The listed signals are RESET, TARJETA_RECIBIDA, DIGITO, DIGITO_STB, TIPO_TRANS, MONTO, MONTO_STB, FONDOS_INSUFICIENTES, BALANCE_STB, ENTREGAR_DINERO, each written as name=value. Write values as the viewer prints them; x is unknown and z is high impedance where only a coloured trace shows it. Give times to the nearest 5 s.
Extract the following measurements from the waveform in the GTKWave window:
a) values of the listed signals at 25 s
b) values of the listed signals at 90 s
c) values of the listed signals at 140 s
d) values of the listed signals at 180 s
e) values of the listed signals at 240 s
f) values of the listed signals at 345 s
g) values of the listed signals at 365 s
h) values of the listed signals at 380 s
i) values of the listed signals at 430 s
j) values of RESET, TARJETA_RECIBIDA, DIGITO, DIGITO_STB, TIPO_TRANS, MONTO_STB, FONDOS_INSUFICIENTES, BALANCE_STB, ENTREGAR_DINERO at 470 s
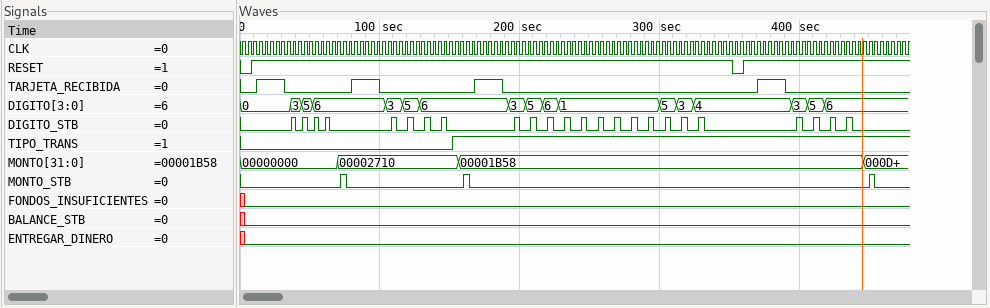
RESET=1, TARJETA_RECIBIDA=1, DIGITO=0, DIGITO_STB=0, TIPO_TRANS=0, MONTO=00000000, MONTO_STB=0, FONDOS_INSUFICIENTES=0, BALANCE_STB=0, ENTREGAR_DINERO=0
RESET=1, TARJETA_RECIBIDA=1, DIGITO=6, DIGITO_STB=0, TIPO_TRANS=0, MONTO=00002710, MONTO_STB=0, FONDOS_INSUFICIENTES=0, BALANCE_STB=0, ENTREGAR_DINERO=0
RESET=1, TARJETA_RECIBIDA=0, DIGITO=6, DIGITO_STB=0, TIPO_TRANS=0, MONTO=00002710, MONTO_STB=0, FONDOS_INSUFICIENTES=0, BALANCE_STB=0, ENTREGAR_DINERO=0
RESET=1, TARJETA_RECIBIDA=1, DIGITO=6, DIGITO_STB=0, TIPO_TRANS=1, MONTO=00001B58, MONTO_STB=0, FONDOS_INSUFICIENTES=0, BALANCE_STB=0, ENTREGAR_DINERO=0
RESET=1, TARJETA_RECIBIDA=0, DIGITO=1, DIGITO_STB=0, TIPO_TRANS=1, MONTO=00001B58, MONTO_STB=0, FONDOS_INSUFICIENTES=0, BALANCE_STB=0, ENTREGAR_DINERO=0
RESET=1, TARJETA_RECIBIDA=0, DIGITO=4, DIGITO_STB=0, TIPO_TRANS=1, MONTO=00001B58, MONTO_STB=0, FONDOS_INSUFICIENTES=0, BALANCE_STB=0, ENTREGAR_DINERO=0
RESET=1, TARJETA_RECIBIDA=0, DIGITO=4, DIGITO_STB=0, TIPO_TRANS=1, MONTO=00001B58, MONTO_STB=0, FONDOS_INSUFICIENTES=0, BALANCE_STB=0, ENTREGAR_DINERO=0
RESET=1, TARJETA_RECIBIDA=1, DIGITO=4, DIGITO_STB=0, TIPO_TRANS=1, MONTO=00001B58, MONTO_STB=0, FONDOS_INSUFICIENTES=0, BALANCE_STB=0, ENTREGAR_DINERO=0
RESET=1, TARJETA_RECIBIDA=0, DIGITO=6, DIGITO_STB=0, TIPO_TRANS=1, MONTO=00001B58, MONTO_STB=0, FONDOS_INSUFICIENTES=0, BALANCE_STB=0, ENTREGAR_DINERO=0
RESET=1, TARJETA_RECIBIDA=0, DIGITO=6, DIGITO_STB=0, TIPO_TRANS=1, MONTO_STB=0, FONDOS_INSUFICIENTES=0, BALANCE_STB=0, ENTREGAR_DINERO=0
